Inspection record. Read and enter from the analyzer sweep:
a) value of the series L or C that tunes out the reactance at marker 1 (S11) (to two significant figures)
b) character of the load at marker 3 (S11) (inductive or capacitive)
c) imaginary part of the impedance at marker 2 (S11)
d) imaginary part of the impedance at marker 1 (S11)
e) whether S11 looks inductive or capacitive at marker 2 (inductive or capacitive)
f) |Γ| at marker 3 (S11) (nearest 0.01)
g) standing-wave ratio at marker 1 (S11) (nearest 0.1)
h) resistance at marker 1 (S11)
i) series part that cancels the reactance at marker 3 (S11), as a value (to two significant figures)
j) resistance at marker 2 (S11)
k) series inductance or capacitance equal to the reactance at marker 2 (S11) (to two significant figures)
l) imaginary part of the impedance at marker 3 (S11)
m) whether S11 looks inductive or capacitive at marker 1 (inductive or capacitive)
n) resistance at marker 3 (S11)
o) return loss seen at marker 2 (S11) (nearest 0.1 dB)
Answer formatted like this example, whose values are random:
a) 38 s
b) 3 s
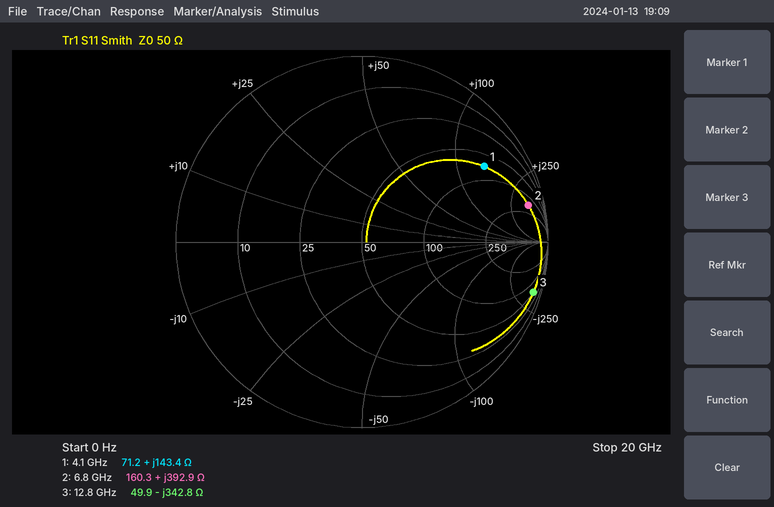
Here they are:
a) 270 fF
b) capacitive
c) +392.9 Ω
d) +143.4 Ω
e) inductive
f) 0.96
g) 7.8
h) 71.2 Ω
i) 4.3 nH
j) 160.3 Ω
k) 9.2 nH
l) -342.8 Ω
m) inductive
n) 49.9 Ω
o) 0.8 dB
